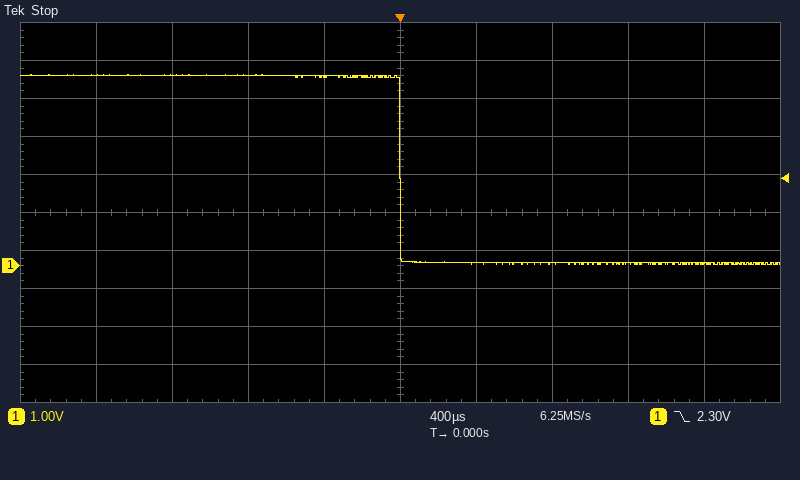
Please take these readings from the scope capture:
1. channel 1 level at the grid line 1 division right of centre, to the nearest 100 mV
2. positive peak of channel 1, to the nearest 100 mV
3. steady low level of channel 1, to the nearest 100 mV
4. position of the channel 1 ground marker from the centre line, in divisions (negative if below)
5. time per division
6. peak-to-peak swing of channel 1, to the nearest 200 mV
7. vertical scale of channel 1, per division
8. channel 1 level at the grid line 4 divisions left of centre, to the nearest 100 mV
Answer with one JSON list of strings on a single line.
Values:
["100 mV", "5.0 V", "100 mV", "-1.4 div", "400 µs", "5.0 V", "1 V", "5.0 V"]
